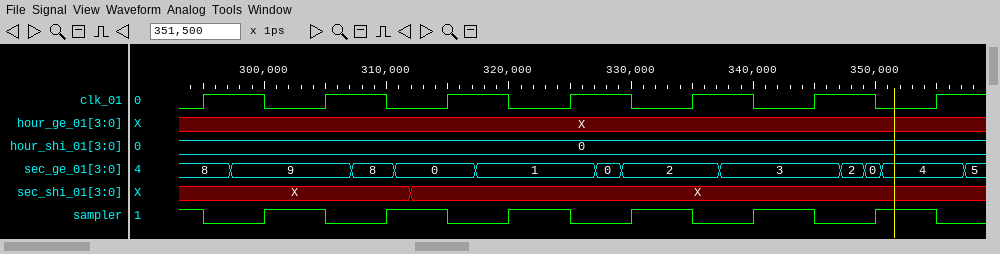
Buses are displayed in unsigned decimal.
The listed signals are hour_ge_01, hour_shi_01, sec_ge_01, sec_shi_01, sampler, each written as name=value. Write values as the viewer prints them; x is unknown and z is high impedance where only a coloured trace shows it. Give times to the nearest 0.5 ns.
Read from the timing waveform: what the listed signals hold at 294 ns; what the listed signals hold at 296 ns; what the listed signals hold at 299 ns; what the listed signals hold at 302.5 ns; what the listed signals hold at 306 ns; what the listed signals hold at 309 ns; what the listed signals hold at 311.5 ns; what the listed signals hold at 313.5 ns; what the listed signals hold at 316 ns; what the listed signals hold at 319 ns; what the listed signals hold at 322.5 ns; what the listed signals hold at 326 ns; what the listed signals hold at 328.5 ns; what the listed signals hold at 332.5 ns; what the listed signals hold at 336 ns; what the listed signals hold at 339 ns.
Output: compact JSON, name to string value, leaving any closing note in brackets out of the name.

{"what the listed signals hold at 294 ns": "hour_ge_01=X, hour_shi_01=0, sec_ge_01=8, sec_shi_01=X, sampler=1", "what the listed signals hold at 296 ns": "hour_ge_01=X, hour_shi_01=0, sec_ge_01=8, sec_shi_01=X, sampler=0", "what the listed signals hold at 299 ns": "hour_ge_01=X, hour_shi_01=0, sec_ge_01=9, sec_shi_01=X, sampler=0", "what the listed signals hold at 302.5 ns": "hour_ge_01=X, hour_shi_01=0, sec_ge_01=9, sec_shi_01=X, sampler=1", "what the listed signals hold at 306 ns": "hour_ge_01=X, hour_shi_01=0, sec_ge_01=9, sec_shi_01=X, sampler=0", "what the listed signals hold at 309 ns": "hour_ge_01=X, hour_shi_01=0, sec_ge_01=8, sec_shi_01=X, sampler=0", "what the listed signals hold at 311.5 ns": "hour_ge_01=X, hour_shi_01=0, sec_ge_01=0, sec_shi_01=X, sampler=1", "what the listed signals hold at 313.5 ns": "hour_ge_01=X, hour_shi_01=0, sec_ge_01=0, sec_shi_01=X, sampler=1", "what the listed signals hold at 316 ns": "hour_ge_01=X, hour_shi_01=0, sec_ge_01=0, sec_shi_01=X, sampler=0", "what the listed signals hold at 319 ns": "hour_ge_01=X, hour_shi_01=0, sec_ge_01=1, sec_shi_01=X, sampler=0", "what the listed signals hold at 322.5 ns": "hour_ge_01=X, hour_shi_01=0, sec_ge_01=1, sec_shi_01=X, sampler=1", "what the listed signals hold at 326 ns": "hour_ge_01=X, hour_shi_01=0, sec_ge_01=1, sec_shi_01=X, sampler=0", "what the listed signals hold at 328.5 ns": "hour_ge_01=X, hour_shi_01=0, sec_ge_01=0, sec_shi_01=X, sampler=0", "what the listed signals hold at 332.5 ns": "hour_ge_01=X, hour_shi_01=0, sec_ge_01=2, sec_shi_01=X, sampler=1", "what the listed signals hold at 336 ns": "hour_ge_01=X, hour_shi_01=0, sec_ge_01=2, sec_shi_01=X, sampler=0", "what the listed signals hold at 339 ns": "hour_ge_01=X, hour_shi_01=0, sec_ge_01=3, sec_shi_01=X, sampler=0"}
